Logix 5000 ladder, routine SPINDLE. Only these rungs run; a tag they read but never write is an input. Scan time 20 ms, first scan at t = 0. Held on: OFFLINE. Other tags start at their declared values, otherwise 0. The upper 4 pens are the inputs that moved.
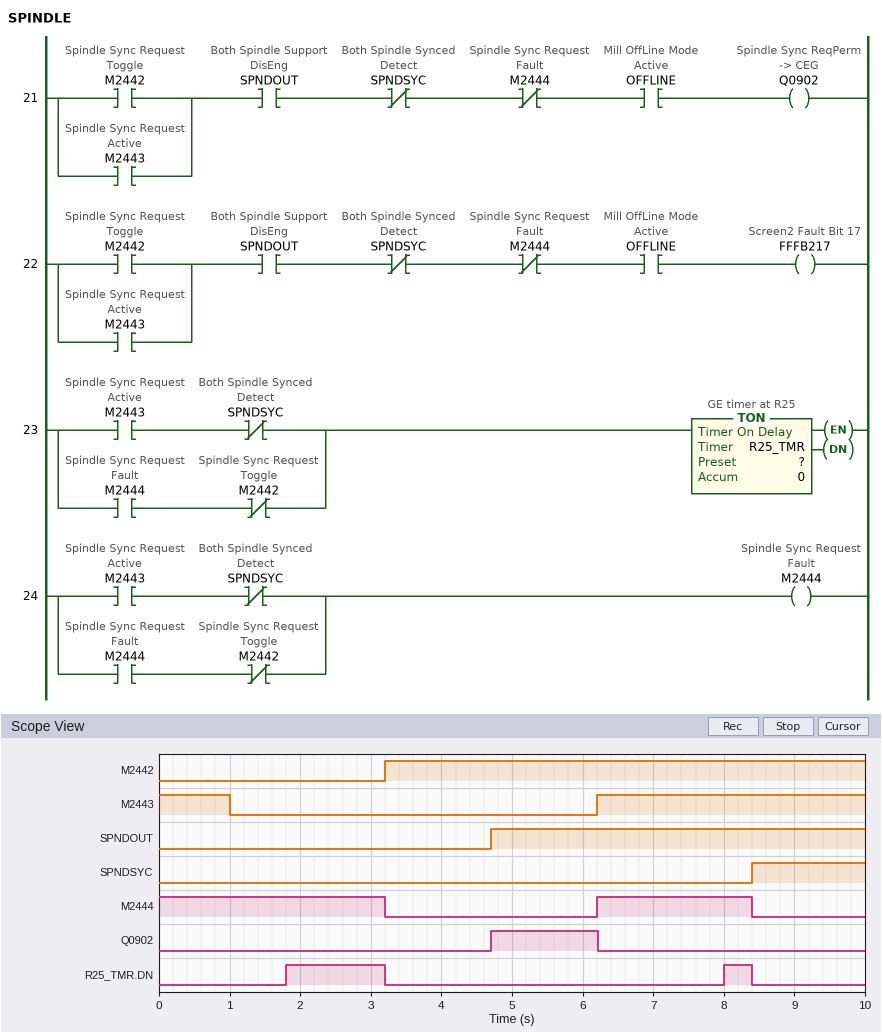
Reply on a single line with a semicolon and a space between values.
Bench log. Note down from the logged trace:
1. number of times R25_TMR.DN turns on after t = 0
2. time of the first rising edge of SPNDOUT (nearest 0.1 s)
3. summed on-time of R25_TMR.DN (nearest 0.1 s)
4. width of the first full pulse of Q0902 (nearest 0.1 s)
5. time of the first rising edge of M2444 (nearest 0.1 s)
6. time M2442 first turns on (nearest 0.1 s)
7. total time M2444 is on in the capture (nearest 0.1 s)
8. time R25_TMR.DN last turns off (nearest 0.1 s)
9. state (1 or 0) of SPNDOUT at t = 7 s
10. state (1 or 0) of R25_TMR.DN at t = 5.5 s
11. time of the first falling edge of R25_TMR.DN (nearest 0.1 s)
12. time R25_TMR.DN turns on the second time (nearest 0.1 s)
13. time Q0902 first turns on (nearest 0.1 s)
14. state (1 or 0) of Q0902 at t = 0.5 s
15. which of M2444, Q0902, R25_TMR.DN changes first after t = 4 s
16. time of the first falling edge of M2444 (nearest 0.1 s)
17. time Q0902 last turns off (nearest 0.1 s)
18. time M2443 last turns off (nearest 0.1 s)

2; 4.7 s; 1.8 s; 1.5 s; 6.2 s; 3.2 s; 5.4 s; 8.4 s; 1; 0; 3.2 s; 8.0 s; 4.7 s; 0; Q0902; 3.2 s; 6.2 s; 1.0 s
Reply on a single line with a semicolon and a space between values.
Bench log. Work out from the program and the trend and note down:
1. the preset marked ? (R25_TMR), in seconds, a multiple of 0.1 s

1.8 s
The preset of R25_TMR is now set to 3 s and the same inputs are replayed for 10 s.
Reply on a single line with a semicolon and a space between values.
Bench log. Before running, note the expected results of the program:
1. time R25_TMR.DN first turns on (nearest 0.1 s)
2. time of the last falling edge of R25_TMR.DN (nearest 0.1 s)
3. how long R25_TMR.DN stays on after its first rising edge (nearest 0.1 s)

3.0 s; 3.2 s; 0.2 s
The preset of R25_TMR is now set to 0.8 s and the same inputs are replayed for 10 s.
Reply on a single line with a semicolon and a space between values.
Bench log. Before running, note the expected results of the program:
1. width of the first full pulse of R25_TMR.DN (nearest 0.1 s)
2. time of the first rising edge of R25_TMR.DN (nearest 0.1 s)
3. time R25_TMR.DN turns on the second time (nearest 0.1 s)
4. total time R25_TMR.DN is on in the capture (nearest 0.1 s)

2.4 s; 0.8 s; 7.0 s; 3.8 s
